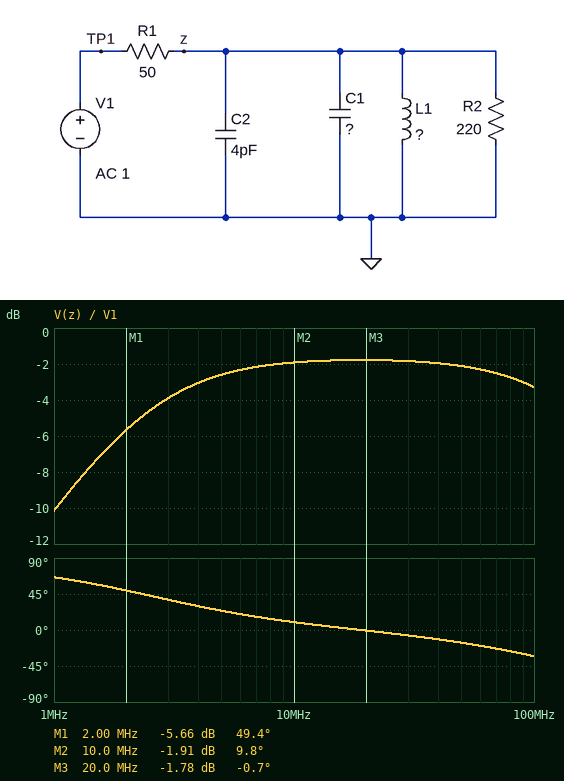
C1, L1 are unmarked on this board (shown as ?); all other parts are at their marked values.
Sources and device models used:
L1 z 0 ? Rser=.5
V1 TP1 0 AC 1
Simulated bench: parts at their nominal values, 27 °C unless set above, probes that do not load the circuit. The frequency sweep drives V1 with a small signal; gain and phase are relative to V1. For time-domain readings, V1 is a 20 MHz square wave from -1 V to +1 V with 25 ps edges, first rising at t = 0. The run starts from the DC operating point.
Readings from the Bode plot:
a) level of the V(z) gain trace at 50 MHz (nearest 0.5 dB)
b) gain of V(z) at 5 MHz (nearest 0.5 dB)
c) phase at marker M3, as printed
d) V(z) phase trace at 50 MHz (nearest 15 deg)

-2.0 dB
-2.5 dB
-0.7 deg
-15 deg
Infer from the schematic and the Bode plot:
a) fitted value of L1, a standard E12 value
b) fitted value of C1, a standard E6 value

2.7 µH
22 pF
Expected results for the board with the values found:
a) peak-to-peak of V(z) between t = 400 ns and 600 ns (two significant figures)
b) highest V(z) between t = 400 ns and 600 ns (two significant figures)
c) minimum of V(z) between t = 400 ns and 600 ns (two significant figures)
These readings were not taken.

1.8 V
910 mV
-910 mV
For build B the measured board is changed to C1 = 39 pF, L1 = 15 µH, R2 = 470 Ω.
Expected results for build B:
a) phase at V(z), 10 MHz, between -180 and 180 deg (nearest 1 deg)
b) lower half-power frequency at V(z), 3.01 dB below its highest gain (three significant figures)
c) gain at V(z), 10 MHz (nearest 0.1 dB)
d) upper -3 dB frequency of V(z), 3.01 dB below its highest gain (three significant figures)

-4 deg
482 kHz
-0.9 dB
82.4 MHz
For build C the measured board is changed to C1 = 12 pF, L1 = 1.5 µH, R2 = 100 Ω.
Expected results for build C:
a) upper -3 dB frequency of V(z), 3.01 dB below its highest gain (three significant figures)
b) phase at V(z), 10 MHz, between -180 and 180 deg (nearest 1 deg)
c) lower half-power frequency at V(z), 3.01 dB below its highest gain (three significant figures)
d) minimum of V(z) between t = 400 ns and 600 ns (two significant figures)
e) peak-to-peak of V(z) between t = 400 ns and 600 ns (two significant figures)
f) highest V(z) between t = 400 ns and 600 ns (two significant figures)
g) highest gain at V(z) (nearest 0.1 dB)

302 MHz
18 deg
3.55 MHz
-810 mV
1.6 V
810 mV
-3.5 dB
